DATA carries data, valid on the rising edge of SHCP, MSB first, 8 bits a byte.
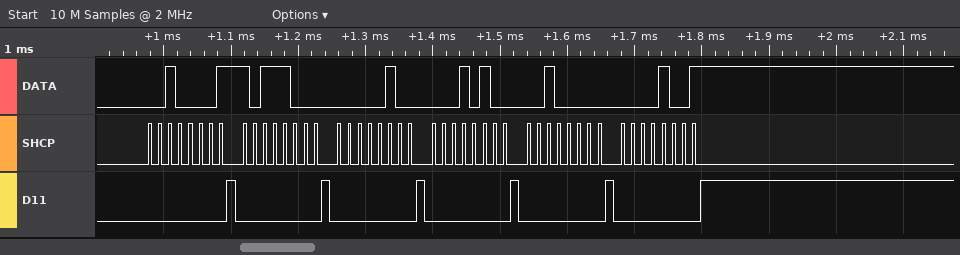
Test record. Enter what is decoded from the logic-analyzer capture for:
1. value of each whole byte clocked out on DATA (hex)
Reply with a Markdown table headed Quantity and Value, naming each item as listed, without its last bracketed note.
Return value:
| Quantity | Value |
|---|---|
| value of each whole byte clocked out on DATA | 21 B8 04 14 20 09 |
